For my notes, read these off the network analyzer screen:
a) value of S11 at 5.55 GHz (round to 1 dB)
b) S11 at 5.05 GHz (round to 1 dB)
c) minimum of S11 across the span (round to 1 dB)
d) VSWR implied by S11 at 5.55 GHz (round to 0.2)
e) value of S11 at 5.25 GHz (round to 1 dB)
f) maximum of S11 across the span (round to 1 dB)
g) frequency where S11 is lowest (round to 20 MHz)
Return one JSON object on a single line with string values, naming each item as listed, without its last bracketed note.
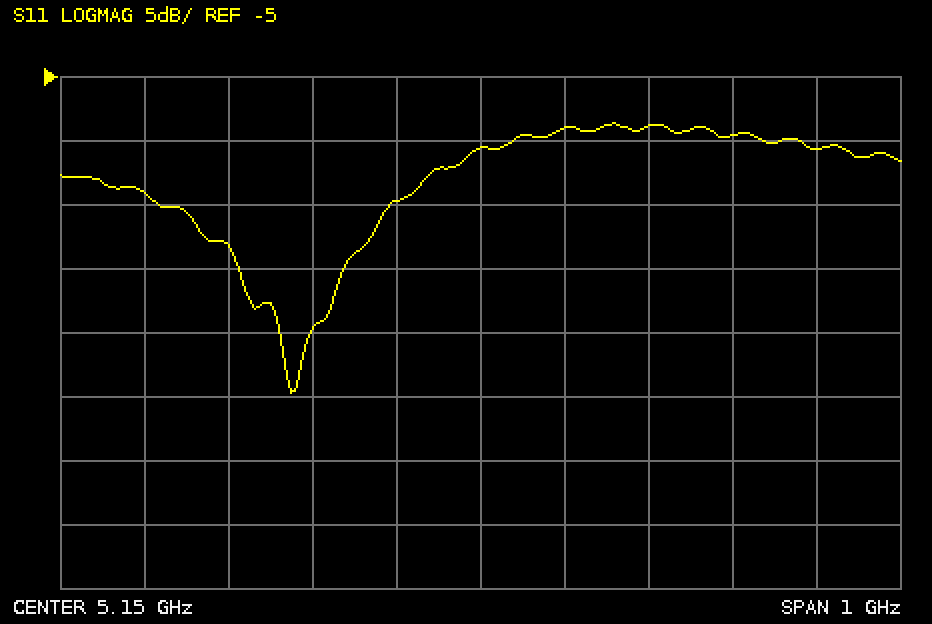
{"value of S11 at 5.55 GHz": "-11 dB", "S11 at 5.05 GHz": "-15 dB", "minimum of S11 across the span": "-30 dB", "VSWR implied by S11 at 5.55 GHz": "1.8", "value of S11 at 5.25 GHz": "-9 dB", "maximum of S11 across the span": "-9 dB", "frequency where S11 is lowest": "4.92 GHz"}
